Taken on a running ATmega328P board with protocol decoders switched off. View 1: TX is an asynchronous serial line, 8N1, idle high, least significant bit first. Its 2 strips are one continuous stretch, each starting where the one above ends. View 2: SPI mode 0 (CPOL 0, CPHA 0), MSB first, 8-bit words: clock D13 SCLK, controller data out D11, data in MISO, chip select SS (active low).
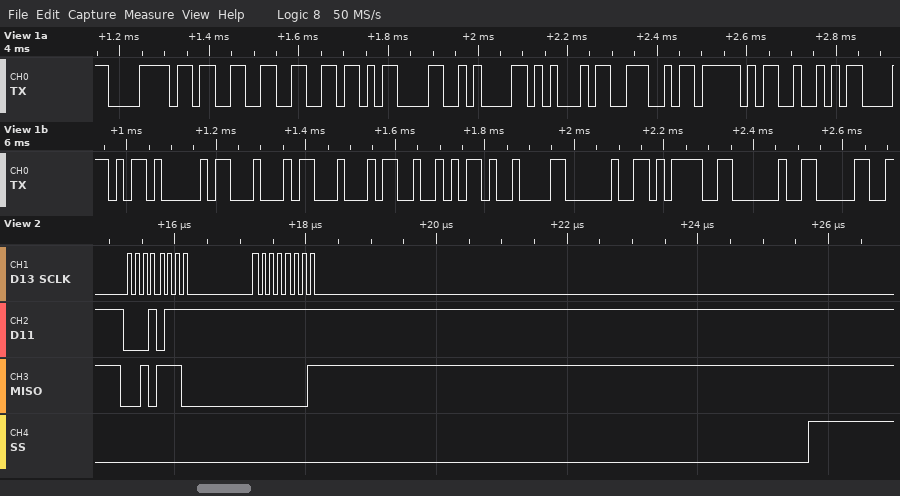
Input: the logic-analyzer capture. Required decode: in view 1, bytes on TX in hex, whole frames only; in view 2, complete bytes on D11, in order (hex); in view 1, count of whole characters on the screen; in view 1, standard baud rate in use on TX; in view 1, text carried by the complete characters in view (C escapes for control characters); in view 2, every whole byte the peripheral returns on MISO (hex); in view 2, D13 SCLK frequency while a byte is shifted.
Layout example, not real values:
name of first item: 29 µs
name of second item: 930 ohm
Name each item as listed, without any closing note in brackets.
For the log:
in view 1, bytes on TX in hex, whole frames only: 78 33 66 0D 0A 45 4E 5F 52 58 41 44 44 52 09 20 3D 20 30
in view 2, complete bytes on D11, in order: 17 FF
in view 1, count of whole characters on the screen: 19
in view 1, standard baud rate in use on TX: 57600 baud
in view 1, text carried by the complete characters in view: "x3f\r\nEN_RXADDR\t = 0"
in view 2, every whole byte the peripheral returns on MISO: 2E 01
in view 2, D13 SCLK frequency while a byte is shifted: 8 MHz
